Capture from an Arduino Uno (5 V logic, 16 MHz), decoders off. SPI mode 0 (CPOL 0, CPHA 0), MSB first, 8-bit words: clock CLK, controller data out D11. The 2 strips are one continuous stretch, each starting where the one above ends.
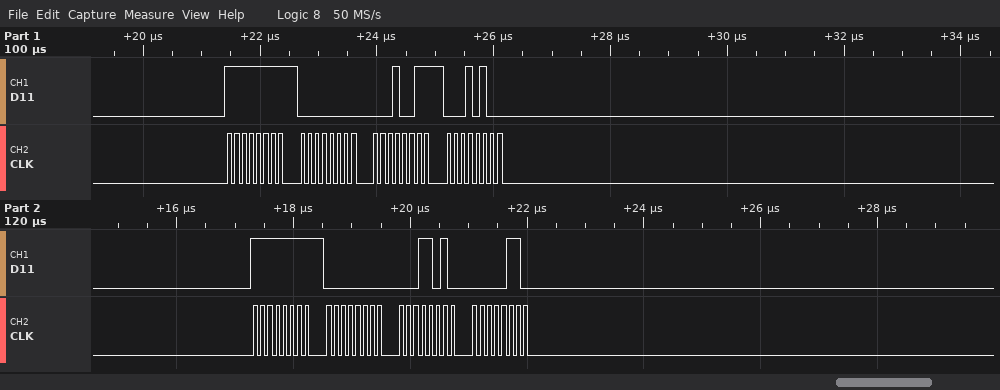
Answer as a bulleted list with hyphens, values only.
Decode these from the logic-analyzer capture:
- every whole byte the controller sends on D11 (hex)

- 0xFF 0x00 0x13 0x14 0xFF 0x00 0x1A 0x06
